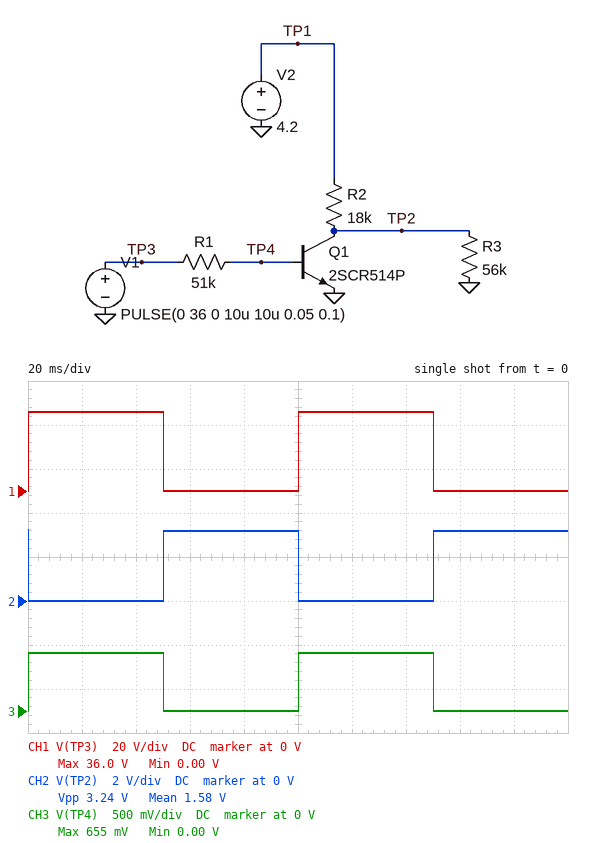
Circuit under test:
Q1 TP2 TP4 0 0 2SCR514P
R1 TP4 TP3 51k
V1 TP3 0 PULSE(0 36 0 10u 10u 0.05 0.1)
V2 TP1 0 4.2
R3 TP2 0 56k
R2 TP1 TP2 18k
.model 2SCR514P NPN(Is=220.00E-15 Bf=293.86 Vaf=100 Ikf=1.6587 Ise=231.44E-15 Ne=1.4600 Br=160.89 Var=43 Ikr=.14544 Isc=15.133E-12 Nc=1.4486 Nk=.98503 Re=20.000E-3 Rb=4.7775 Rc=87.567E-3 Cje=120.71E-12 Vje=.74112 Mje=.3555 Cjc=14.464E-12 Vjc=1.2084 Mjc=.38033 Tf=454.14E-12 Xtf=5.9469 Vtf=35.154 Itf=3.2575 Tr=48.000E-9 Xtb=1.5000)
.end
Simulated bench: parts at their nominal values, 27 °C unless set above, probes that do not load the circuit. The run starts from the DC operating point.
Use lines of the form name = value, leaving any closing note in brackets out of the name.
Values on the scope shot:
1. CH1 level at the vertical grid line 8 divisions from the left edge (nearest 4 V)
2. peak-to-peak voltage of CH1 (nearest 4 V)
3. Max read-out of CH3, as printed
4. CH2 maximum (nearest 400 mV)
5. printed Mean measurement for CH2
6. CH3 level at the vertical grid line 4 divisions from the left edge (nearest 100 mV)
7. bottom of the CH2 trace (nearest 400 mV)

CH1 level at the vertical grid line 8 divisions from the left edge = 0 V
peak-to-peak voltage of CH1 = 36 V
Max read-out of CH3, as printed = 655 mV
CH2 maximum = 3.2 V
printed Mean measurement for CH2 = 1.58 V
CH3 level at the vertical grid line 4 divisions from the left edge = 0 V
bottom of the CH2 trace = 0 V
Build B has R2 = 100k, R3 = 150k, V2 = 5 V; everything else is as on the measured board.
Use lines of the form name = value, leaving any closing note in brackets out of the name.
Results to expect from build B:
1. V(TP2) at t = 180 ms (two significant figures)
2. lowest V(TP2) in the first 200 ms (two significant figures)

V(TP2) at t = 180 ms = 3.0 V
lowest V(TP2) in the first 200 ms = 1.1 mV
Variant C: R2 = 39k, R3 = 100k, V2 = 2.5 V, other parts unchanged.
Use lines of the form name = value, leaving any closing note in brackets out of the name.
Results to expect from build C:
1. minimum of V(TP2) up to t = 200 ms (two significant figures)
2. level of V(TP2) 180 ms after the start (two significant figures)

minimum of V(TP2) up to t = 200 ms = 1.1 mV
level of V(TP2) 180 ms after the start = 1.8 V
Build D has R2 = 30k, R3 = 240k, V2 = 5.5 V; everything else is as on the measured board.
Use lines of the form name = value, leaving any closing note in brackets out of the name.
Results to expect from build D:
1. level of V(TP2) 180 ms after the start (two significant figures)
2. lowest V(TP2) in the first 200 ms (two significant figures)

level of V(TP2) 180 ms after the start = 4.9 V
lowest V(TP2) in the first 200 ms = 1.4 mV
